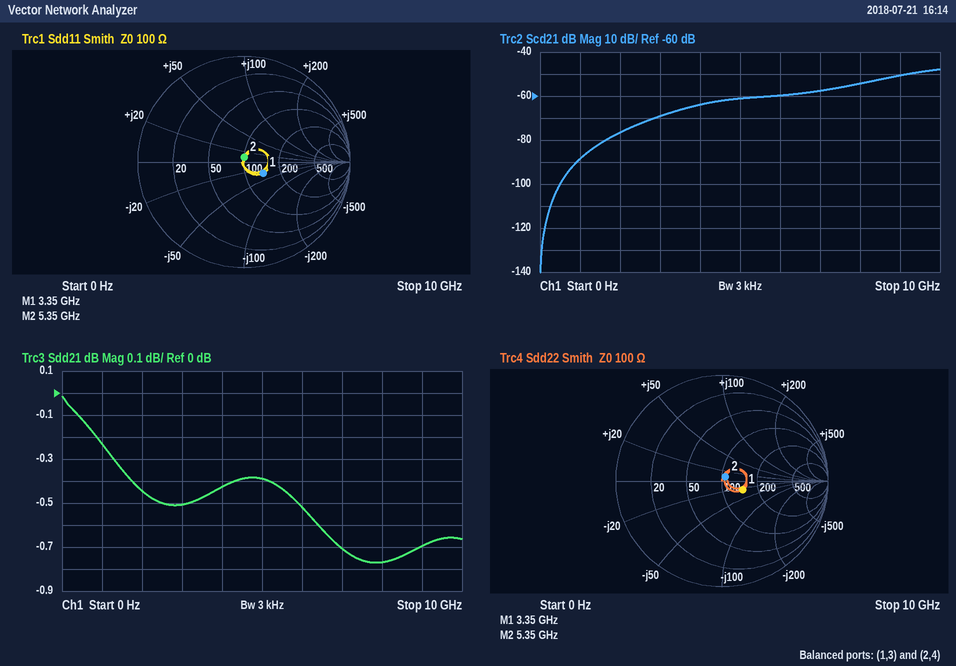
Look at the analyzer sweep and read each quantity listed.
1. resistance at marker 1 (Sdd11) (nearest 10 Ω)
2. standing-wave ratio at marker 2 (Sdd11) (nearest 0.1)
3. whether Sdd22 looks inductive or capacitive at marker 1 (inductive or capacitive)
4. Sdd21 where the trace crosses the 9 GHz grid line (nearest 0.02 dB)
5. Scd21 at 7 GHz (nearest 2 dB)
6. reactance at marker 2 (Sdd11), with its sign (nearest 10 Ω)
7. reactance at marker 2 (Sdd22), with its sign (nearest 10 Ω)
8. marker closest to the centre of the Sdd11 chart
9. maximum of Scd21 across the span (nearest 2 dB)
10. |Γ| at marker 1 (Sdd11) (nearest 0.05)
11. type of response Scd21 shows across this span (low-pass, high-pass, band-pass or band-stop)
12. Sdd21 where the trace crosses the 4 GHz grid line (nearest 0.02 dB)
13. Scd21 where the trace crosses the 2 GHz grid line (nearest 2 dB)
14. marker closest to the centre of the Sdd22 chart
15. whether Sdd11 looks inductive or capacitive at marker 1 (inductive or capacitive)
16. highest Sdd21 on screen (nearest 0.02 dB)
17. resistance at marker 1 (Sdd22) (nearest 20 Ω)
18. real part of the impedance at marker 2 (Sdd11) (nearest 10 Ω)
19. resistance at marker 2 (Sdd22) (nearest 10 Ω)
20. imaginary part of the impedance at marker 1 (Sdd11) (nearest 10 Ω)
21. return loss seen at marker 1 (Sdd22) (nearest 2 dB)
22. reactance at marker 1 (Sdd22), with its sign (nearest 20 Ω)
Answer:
140 Ω
1.1
capacitive
-0.70 dB
-58 dB
+10 Ω
+10 Ω
marker 2
-48 dB
0.20
high-pass
-0.42 dB
-76 dB
marker 2
capacitive
-0.02 dB
140 Ω
100 Ω
110 Ω
-30 Ω
14 dB
-20 Ω
